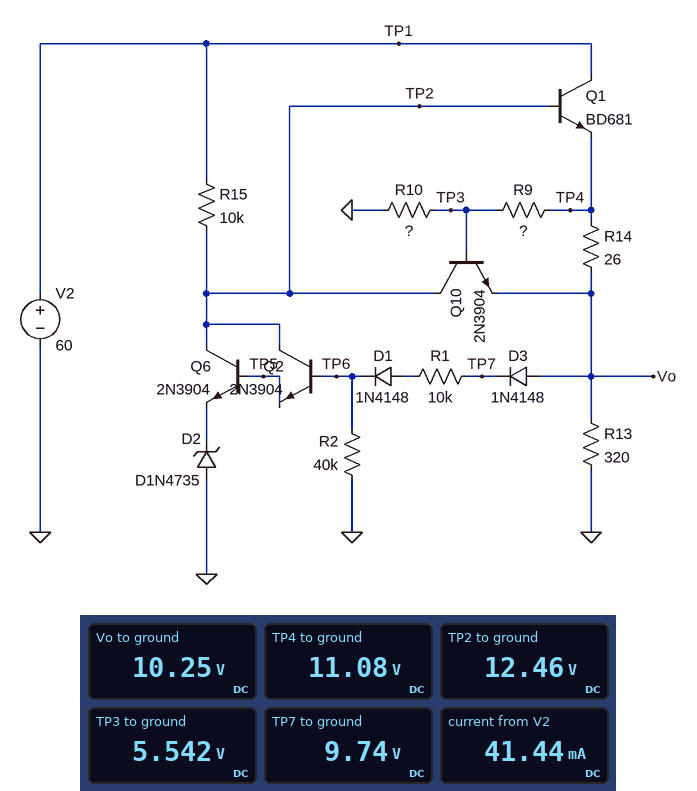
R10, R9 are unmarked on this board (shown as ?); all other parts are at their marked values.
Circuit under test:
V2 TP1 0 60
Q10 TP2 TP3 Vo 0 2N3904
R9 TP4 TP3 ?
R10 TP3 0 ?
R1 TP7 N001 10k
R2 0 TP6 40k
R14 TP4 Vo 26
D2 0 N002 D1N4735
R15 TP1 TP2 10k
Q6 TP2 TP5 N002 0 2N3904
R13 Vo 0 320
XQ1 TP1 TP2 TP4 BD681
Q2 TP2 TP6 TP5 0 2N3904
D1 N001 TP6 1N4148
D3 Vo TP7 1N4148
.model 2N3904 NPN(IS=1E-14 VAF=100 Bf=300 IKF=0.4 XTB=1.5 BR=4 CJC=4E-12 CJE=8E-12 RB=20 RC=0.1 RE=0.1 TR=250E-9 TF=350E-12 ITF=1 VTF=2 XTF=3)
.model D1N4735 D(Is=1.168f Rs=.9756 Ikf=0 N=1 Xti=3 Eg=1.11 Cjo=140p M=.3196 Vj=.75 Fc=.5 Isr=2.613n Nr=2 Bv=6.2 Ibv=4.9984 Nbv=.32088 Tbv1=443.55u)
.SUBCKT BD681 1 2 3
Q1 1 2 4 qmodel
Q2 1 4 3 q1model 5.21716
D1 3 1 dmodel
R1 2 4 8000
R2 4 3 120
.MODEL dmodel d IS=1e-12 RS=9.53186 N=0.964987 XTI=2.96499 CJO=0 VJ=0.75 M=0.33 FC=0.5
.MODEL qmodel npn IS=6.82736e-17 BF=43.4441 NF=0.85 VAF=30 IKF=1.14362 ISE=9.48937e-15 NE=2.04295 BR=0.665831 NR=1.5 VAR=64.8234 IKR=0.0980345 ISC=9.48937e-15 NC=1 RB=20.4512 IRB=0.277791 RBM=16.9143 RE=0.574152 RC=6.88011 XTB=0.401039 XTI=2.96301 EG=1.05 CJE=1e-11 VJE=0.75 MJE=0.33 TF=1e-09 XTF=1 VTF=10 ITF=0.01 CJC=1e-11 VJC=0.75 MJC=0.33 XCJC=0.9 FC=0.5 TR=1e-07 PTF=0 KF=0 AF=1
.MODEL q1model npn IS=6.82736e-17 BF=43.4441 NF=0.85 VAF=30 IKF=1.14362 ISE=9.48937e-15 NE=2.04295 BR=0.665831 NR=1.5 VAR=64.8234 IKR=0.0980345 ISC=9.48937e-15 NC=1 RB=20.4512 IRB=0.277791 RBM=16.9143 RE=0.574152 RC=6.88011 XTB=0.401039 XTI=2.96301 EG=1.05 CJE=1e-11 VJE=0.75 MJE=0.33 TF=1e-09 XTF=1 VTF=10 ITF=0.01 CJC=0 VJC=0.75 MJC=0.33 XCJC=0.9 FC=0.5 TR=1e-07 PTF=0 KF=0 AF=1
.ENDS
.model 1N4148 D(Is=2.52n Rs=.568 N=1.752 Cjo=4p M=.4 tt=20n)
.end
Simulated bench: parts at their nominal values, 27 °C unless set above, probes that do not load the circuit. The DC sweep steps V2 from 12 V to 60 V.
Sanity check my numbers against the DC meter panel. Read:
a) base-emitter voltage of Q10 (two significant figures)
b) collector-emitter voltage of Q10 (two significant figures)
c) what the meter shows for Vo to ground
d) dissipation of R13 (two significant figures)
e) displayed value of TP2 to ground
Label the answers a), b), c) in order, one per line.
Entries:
a) -4.7 V
b) 2.2 V
c) 10.25 V
d) 330 mW
e) 12.46 V
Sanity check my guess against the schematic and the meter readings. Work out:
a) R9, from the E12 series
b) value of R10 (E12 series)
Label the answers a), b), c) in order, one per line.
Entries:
a) 1.2 kΩ
b) 1.2 kΩ
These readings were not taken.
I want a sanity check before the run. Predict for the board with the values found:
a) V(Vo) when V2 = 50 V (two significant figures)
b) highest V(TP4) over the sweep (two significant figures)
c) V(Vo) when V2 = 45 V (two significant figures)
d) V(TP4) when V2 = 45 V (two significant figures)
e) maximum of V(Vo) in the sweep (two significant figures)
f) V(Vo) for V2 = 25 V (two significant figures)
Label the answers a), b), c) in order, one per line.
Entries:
a) 10 V
b) 11 V
c) 10 V
d) 11 V
e) 10 V
f) 10 V
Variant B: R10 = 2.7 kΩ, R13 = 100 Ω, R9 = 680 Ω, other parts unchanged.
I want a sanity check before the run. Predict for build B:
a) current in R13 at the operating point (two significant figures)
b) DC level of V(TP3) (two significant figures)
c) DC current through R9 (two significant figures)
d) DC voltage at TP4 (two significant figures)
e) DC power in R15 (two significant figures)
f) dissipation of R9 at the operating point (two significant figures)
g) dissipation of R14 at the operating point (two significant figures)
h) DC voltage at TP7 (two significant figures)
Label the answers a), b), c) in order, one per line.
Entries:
a) 100 mA
b) 10 V
c) 3.8 mA
d) 13 V
e) 210 mW
f) 9.9 mW
g) 270 mW
h) 9.7 V
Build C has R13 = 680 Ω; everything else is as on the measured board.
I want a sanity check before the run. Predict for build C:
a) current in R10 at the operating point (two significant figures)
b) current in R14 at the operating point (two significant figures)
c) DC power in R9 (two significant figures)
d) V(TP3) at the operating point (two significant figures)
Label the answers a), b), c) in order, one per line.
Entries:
a) 4.4 mA
b) 15 mA
c) 24 mW
d) 5.3 V
